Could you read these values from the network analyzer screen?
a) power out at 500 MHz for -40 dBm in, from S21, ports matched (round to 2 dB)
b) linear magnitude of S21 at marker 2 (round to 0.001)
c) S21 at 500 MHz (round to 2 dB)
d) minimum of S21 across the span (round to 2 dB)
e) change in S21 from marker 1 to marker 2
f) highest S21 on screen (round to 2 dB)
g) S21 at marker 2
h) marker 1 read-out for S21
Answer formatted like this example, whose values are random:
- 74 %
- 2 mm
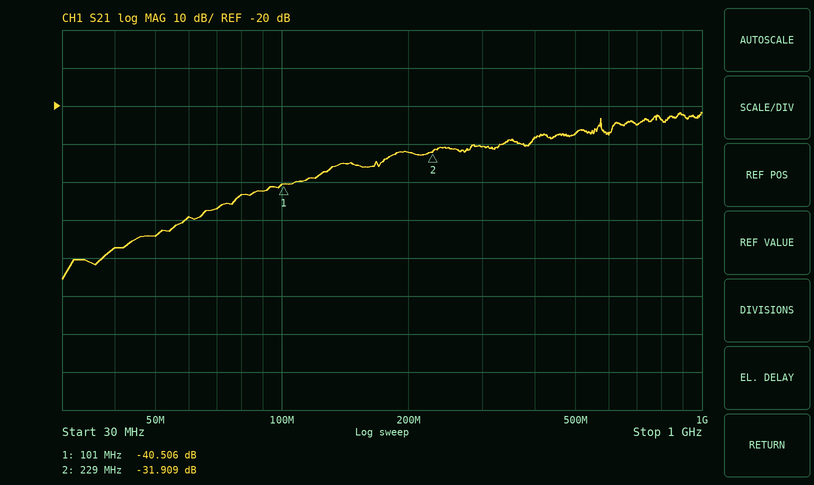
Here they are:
- -68 dBm
- 0.025
- -28 dB
- -66 dB
- 8.597 dB
- -22 dB
- -31.909 dB
- -40.506 dB
